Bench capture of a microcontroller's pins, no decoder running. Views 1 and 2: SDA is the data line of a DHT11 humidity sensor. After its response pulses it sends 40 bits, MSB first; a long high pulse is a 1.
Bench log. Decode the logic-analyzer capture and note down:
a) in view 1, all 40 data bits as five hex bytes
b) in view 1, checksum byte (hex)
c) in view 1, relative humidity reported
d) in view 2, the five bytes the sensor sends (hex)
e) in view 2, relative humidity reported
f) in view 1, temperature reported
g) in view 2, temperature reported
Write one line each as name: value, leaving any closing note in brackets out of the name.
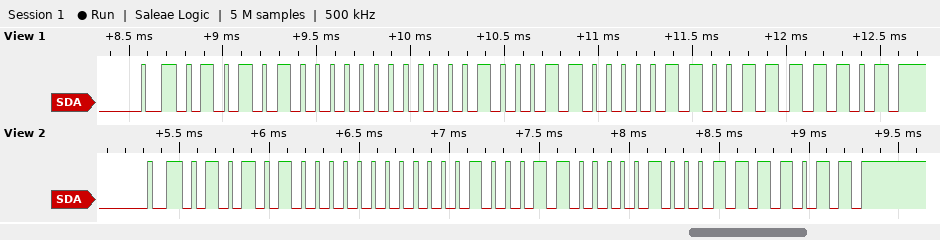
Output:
in view 1, all 40 data bits as five hex bytes: 54 00 23 06 7D
in view 1, checksum byte: 0x7D
in view 1, relative humidity reported: 84 %
in view 2, the five bytes the sensor sends: 54 00 23 04 7B
in view 2, relative humidity reported: 84 %
in view 1, temperature reported: 35.6 °C
in view 2, temperature reported: 35.4 °C
